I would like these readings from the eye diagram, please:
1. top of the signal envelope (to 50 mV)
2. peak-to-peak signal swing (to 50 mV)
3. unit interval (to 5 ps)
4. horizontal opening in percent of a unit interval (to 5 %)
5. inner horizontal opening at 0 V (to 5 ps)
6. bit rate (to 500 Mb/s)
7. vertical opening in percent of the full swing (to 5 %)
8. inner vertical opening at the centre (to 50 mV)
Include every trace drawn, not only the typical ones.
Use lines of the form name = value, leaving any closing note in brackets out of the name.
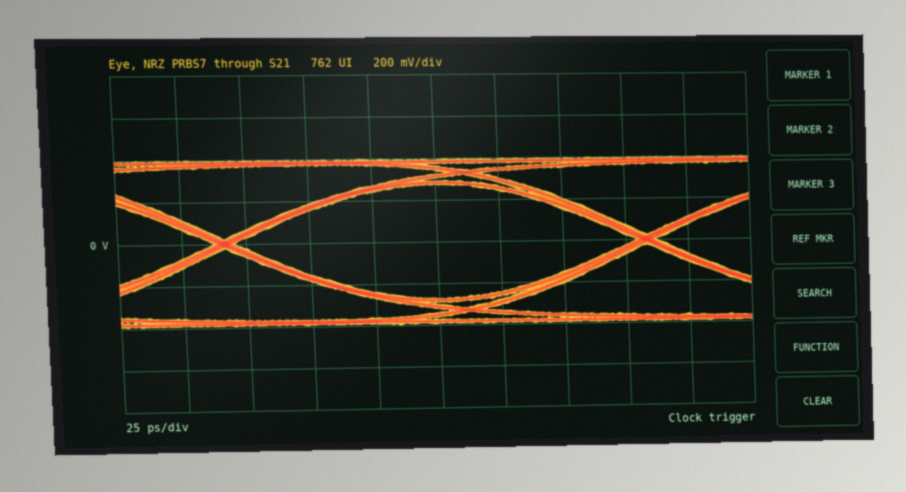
top of the signal envelope = 400 mV
peak-to-peak signal swing = 800 mV
unit interval = 165 ps
horizontal opening in percent of a unit interval = 95 %
inner horizontal opening at 0 V = 160 ps
bit rate = 6.0 Gb/s
vertical opening in percent of the full swing = 70 %
inner vertical opening at the centre = 550 mV
